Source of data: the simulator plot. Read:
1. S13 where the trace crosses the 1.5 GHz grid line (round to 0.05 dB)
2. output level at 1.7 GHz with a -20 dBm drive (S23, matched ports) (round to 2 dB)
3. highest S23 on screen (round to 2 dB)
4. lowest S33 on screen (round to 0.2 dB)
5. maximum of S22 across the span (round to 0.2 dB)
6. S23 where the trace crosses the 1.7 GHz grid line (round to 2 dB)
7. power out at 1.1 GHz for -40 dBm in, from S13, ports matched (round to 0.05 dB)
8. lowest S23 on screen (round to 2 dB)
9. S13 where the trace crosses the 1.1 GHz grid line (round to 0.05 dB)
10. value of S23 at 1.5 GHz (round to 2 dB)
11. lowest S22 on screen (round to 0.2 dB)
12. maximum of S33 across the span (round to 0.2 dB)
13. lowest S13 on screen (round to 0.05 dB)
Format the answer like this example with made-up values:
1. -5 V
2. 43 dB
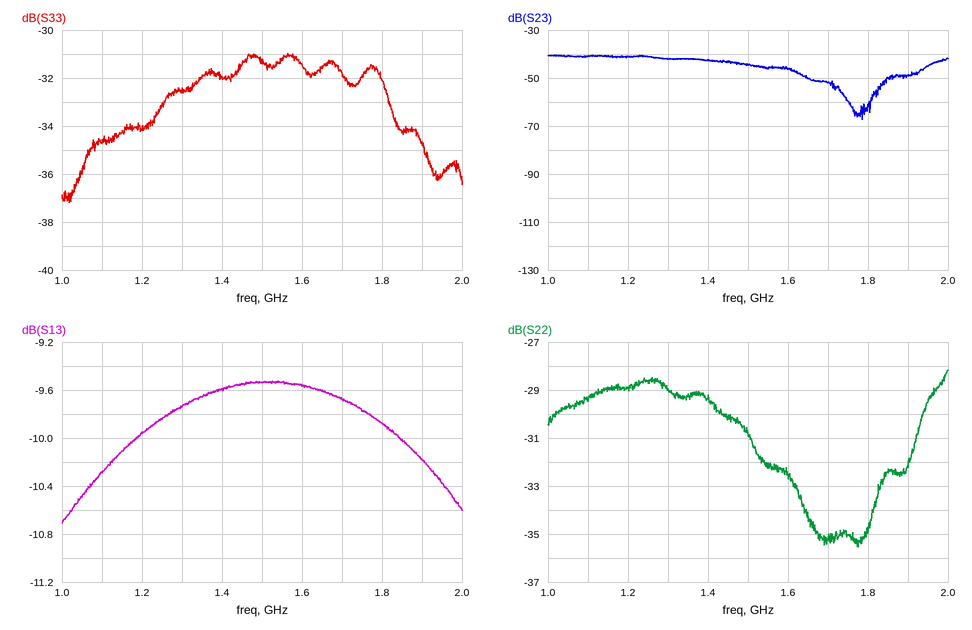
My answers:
1. -9.55 dB
2. -72 dBm
3. -40 dB
4. -37.2 dB
5. -28.2 dB
6. -52 dB
7. -50.30 dBm
8. -68 dB
9. -10.30 dB
10. -44 dB
11. -35.6 dB
12. -31.0 dB
13. -10.70 dB
